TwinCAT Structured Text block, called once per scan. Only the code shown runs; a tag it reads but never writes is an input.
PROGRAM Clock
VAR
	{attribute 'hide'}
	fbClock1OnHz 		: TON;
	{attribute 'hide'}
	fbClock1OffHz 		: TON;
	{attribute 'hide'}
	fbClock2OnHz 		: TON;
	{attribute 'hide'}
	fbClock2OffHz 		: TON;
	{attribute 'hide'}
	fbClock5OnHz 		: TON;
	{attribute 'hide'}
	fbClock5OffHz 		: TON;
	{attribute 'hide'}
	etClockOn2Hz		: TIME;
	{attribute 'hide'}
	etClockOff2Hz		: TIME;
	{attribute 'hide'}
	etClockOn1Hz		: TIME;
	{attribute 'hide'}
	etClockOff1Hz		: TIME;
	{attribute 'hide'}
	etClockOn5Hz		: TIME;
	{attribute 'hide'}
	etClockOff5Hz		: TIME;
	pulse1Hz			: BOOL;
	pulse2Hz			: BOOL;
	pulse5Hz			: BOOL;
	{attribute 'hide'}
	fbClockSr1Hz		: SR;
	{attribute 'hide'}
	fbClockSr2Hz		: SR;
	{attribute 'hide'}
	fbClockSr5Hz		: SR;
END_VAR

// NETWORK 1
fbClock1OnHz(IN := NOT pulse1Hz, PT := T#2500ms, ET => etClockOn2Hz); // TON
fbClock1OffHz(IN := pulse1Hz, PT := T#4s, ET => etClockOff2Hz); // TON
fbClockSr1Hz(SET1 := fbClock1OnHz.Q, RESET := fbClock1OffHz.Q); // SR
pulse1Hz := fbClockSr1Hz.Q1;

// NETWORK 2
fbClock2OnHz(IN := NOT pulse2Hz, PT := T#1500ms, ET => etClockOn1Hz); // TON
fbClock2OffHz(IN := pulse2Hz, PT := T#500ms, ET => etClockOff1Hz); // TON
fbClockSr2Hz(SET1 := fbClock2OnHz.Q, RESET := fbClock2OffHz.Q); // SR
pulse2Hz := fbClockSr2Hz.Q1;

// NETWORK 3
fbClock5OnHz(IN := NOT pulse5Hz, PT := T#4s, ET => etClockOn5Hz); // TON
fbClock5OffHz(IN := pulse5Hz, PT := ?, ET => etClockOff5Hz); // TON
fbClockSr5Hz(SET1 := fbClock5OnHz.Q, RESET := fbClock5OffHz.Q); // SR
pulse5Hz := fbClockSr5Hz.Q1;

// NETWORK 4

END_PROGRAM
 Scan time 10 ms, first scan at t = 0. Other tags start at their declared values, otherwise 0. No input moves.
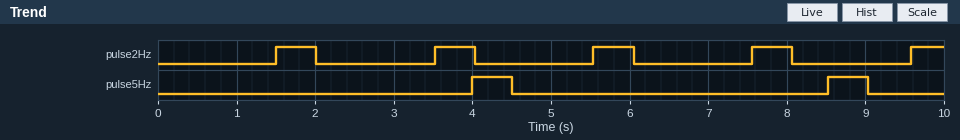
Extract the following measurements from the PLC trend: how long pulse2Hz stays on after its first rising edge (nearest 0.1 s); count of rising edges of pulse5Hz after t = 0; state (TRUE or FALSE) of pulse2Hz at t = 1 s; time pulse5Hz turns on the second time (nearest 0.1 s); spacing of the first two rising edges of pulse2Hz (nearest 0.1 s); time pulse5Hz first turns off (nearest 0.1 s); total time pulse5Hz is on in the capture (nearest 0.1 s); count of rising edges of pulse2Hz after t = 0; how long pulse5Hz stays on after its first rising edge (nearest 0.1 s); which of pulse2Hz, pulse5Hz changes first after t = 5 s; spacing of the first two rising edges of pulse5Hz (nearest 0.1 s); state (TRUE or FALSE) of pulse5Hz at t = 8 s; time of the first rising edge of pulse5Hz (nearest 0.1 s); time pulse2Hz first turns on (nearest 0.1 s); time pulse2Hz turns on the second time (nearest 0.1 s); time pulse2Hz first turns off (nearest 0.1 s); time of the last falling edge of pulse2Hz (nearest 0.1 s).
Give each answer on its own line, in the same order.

0.5 s
2
FALSE
8.5 s
2.0 s
4.5 s
1.0 s
5
0.5 s
pulse2Hz
4.5 s
FALSE
4.0 s
1.5 s
3.5 s
2.0 s
8.1 s
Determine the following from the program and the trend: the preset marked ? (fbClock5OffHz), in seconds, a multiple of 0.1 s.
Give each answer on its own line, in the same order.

0.5 s
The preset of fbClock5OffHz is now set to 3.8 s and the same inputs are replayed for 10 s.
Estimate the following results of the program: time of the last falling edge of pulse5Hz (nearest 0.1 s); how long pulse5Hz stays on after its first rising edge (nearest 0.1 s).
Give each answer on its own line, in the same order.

7.8 s
3.8 s
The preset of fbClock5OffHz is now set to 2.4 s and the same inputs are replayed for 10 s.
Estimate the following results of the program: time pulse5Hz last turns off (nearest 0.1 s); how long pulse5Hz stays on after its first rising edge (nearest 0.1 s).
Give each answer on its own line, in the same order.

6.4 s
2.4 s
